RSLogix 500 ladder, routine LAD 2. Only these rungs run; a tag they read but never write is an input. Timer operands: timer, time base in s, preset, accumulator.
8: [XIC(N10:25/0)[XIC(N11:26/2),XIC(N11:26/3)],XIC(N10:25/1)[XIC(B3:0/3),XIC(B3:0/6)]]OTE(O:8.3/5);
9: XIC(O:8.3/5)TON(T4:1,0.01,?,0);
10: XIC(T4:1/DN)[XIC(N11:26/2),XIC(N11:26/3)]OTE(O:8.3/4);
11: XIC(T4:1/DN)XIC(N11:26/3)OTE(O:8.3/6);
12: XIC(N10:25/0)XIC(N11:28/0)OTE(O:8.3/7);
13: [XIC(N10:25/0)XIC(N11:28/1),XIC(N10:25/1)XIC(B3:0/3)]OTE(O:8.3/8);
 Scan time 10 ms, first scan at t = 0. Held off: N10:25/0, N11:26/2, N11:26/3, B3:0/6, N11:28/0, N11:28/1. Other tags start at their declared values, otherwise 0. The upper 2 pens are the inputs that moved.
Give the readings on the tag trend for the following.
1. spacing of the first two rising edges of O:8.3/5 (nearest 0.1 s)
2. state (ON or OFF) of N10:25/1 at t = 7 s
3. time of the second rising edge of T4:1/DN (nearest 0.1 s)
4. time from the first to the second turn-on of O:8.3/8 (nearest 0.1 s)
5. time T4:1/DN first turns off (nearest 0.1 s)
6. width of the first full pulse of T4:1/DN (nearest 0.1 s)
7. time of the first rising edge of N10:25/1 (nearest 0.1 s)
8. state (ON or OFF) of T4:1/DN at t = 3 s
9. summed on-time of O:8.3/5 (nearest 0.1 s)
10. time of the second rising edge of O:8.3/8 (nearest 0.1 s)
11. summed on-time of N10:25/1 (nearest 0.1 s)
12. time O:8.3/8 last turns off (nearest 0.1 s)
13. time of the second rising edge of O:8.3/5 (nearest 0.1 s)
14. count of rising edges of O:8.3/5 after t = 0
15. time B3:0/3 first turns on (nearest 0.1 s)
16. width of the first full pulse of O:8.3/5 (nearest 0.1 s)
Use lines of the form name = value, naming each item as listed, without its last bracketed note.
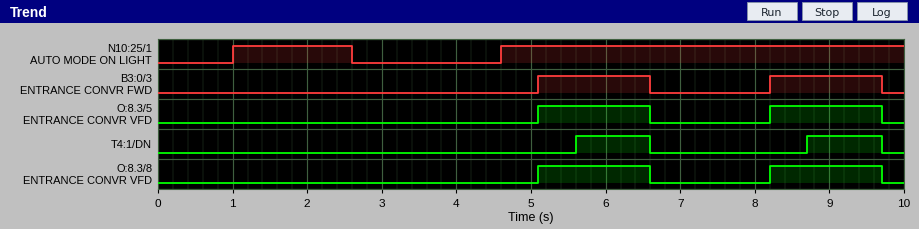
spacing of the first two rising edges of O:8.3/5 = 3.1 s
state (ON or OFF) of N10:25/1 at t = 7 s = ON
time of the second rising edge of T4:1/DN = 8.7 s
time from the first to the second turn-on of O:8.3/8 = 3.1 s
time T4:1/DN first turns off = 6.6 s
width of the first full pulse of T4:1/DN = 1.0 s
time of the first rising edge of N10:25/1 = 1.0 s
state (ON or OFF) of T4:1/DN at t = 3 s = OFF
summed on-time of O:8.3/5 = 3.0 s
time of the second rising edge of O:8.3/8 = 8.2 s
summed on-time of N10:25/1 = 7.0 s
time O:8.3/8 last turns off = 9.7 s
time of the second rising edge of O:8.3/5 = 8.2 s
count of rising edges of O:8.3/5 after t = 0 = 2
time B3:0/3 first turns on = 5.1 s
width of the first full pulse of O:8.3/5 = 1.5 s
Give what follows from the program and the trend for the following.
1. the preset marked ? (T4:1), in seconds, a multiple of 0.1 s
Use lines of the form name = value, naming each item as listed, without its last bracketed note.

the preset marked ? (T4:1), in seconds, a multiple of 0.1 s = 0.5 s
